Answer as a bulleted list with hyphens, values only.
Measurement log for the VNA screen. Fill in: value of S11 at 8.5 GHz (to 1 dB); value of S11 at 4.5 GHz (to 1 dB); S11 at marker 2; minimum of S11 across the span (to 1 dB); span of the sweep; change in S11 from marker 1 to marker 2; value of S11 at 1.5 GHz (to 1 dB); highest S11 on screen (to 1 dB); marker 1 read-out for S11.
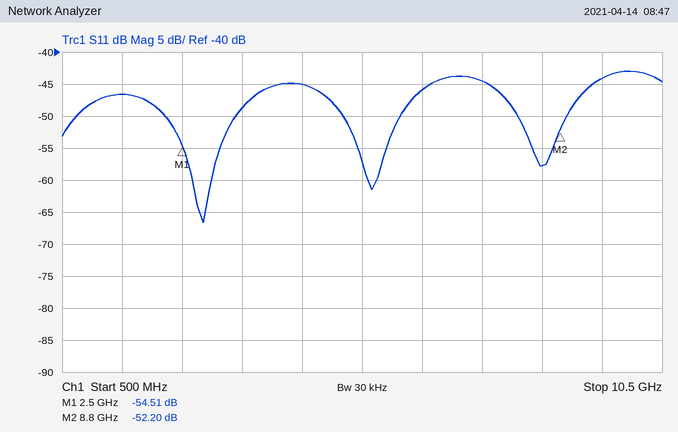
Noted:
- -58 dB
- -45 dB
- -52.20 dB
- -67 dB
- 10 GHz
- 2.31 dB
- -47 dB
- -43 dB
- -54.51 dB
